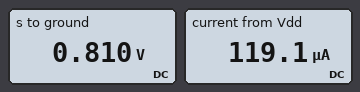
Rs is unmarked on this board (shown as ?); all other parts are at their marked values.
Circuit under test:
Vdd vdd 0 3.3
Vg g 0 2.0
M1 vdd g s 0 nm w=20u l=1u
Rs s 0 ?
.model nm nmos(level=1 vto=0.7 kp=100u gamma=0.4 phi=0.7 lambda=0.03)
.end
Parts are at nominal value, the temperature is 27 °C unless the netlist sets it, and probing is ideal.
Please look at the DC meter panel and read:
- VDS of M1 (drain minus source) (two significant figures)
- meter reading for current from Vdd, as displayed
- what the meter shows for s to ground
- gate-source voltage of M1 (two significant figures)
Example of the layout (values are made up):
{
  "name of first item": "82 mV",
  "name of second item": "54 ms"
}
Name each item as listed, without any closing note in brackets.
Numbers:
{
  "VDS of M1 (drain minus source)": "2.5 V",
  "meter reading for current from Vdd, as displayed": "119.1 µA",
  "what the meter shows for s to ground": "0.810 V",
  "gate-source voltage of M1": "1.2 V"
}
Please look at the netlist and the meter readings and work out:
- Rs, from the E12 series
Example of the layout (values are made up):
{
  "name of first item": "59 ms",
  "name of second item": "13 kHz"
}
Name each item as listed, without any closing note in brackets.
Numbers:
{
  "Rs, from the E12 series": "6.8 kΩ"
}
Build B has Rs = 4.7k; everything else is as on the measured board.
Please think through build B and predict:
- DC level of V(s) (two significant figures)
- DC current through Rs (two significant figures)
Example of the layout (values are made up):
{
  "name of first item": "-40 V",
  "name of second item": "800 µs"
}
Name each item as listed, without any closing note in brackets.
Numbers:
{
  "DC level of V(s)": "760 mV",
  "DC current through Rs": "160 µA"
}
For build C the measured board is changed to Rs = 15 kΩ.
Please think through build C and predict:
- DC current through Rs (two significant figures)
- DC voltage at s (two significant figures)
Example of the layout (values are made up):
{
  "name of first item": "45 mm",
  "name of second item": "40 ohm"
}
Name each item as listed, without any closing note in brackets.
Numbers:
{
  "DC current through Rs": "60 µA",
  "DC voltage at s": "890 mV"
}
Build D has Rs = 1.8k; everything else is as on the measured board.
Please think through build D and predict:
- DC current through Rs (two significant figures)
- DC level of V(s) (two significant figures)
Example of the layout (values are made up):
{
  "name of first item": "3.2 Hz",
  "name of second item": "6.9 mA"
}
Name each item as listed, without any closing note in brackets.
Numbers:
{
  "DC current through Rs": "340 µA",
  "DC level of V(s)": "610 mV"
}
